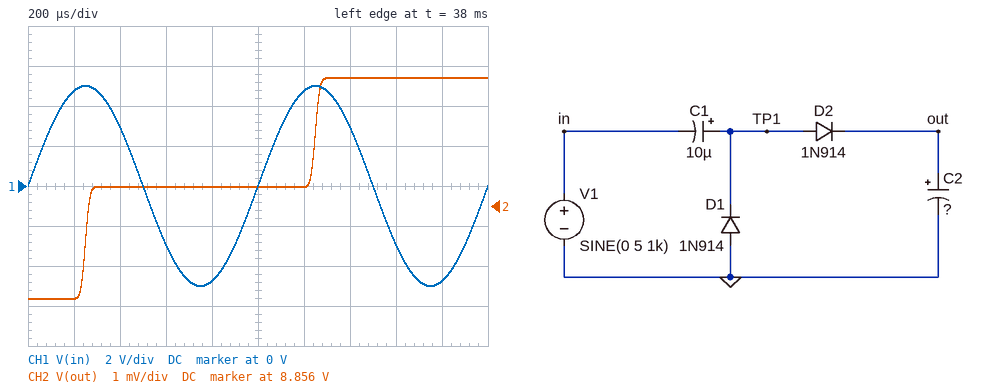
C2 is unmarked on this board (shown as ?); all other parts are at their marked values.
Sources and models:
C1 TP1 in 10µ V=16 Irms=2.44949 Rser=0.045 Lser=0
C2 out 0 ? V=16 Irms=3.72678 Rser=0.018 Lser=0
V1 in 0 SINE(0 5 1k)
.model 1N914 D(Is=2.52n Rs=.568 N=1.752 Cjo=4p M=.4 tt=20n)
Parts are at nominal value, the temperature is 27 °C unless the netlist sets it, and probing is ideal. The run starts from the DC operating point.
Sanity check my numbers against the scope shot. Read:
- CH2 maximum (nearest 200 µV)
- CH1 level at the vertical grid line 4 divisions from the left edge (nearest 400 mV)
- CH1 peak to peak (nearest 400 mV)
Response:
8.8592 V
-4.8 V
10.0 V
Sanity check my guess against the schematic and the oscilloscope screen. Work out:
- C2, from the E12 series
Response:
8.2 µF
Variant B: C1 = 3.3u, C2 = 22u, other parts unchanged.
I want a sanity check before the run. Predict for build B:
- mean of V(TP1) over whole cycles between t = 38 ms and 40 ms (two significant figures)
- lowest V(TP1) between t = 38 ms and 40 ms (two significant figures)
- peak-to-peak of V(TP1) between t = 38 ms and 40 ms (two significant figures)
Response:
4.3 V
-660 mV
10 V
